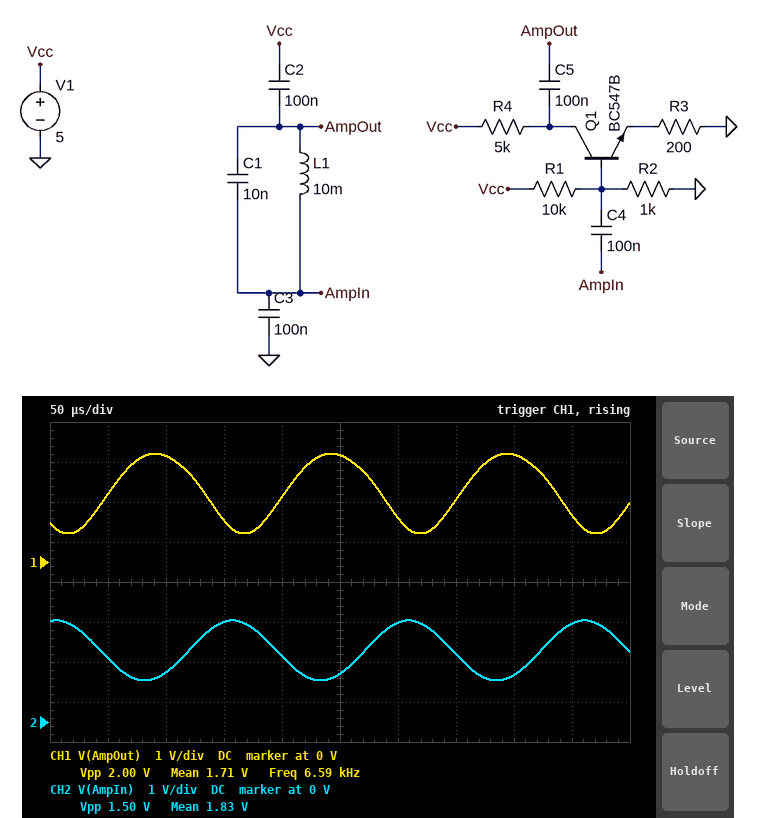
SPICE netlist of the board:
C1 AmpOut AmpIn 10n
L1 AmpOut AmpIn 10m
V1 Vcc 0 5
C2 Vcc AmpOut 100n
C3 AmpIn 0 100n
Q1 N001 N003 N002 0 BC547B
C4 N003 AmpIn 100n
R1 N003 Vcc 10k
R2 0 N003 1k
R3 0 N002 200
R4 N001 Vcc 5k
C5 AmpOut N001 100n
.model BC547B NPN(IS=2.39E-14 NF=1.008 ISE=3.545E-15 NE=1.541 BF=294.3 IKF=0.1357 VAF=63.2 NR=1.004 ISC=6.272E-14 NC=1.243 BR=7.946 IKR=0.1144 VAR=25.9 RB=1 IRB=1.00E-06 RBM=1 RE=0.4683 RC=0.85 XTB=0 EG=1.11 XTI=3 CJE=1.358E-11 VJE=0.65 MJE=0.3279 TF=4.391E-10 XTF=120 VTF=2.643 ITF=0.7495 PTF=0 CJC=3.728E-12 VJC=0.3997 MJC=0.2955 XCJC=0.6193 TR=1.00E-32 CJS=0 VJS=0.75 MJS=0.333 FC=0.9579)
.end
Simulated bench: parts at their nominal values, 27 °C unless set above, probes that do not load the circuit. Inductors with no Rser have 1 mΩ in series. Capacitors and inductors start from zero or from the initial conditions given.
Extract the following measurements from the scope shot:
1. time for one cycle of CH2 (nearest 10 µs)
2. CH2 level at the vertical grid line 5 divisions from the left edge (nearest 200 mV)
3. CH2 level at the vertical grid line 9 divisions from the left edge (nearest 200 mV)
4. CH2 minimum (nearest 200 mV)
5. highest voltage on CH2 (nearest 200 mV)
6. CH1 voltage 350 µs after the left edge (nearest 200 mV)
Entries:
150 µs
1.2 V
2.4 V
1.0 V
2.6 V
1.6 V
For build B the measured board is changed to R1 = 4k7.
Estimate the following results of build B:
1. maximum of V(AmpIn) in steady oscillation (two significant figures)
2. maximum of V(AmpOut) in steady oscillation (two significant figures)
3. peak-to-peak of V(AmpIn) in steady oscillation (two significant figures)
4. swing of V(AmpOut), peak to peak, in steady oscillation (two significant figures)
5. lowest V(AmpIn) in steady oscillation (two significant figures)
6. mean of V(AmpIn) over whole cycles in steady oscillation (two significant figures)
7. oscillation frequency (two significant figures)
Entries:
2.0 V
2.3 V
660 mV
1.1 V
1.4 V
1.7 V
6.8 kHz
